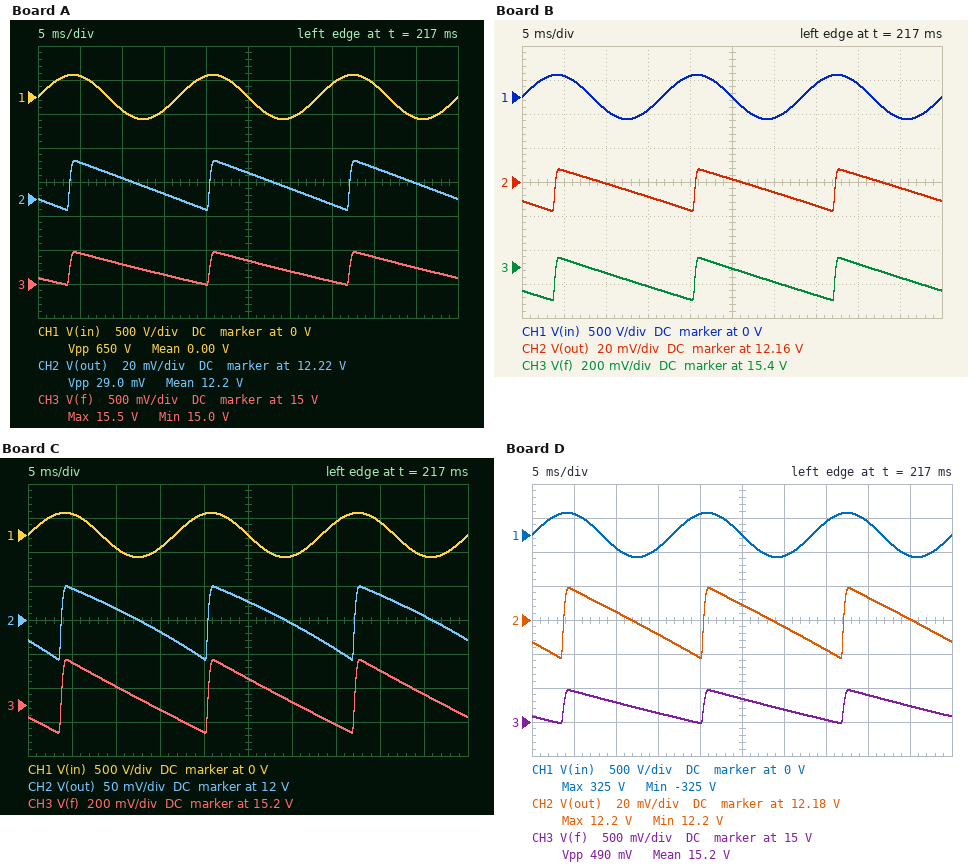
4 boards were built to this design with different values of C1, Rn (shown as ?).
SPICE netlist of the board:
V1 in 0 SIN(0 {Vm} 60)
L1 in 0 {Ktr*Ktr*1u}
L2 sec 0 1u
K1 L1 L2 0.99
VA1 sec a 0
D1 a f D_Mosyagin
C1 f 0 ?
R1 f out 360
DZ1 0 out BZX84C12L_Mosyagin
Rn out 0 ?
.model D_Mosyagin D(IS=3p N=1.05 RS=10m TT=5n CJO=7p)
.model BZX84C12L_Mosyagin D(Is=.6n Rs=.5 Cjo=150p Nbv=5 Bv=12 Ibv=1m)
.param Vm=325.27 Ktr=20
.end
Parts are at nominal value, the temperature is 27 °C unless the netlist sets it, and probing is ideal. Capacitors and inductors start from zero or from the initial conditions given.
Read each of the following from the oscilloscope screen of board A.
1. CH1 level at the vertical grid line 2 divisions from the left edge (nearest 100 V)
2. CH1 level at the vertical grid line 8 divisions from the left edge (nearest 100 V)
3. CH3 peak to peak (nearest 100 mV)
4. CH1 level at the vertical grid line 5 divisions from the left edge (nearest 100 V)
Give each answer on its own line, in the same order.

-200 V
200 V
500 mV
0 V
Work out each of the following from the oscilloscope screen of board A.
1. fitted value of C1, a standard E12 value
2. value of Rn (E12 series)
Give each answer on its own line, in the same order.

270 µF
4.7 kΩ
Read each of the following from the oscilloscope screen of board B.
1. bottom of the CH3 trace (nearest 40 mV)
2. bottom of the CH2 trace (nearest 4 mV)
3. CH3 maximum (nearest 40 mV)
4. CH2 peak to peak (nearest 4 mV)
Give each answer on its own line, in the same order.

15.20 V
12.144 V
15.44 V
24 mV
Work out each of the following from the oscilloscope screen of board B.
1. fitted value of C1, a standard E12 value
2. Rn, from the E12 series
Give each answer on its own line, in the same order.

560 µF
2.2 kΩ
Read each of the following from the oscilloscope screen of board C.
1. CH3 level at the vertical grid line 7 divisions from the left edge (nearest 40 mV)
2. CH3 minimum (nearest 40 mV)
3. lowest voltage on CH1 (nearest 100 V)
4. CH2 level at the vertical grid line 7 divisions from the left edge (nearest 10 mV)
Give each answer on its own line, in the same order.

15.08 V
15.04 V
-300 V
11.96 V
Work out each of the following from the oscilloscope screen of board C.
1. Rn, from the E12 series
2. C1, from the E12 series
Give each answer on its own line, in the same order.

1.5 kΩ
330 µF
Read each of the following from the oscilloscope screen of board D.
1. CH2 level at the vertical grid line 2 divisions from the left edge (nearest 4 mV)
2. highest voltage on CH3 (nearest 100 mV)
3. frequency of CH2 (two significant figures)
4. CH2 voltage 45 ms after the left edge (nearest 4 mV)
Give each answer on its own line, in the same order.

12.184 V
15.5 V
60 Hz
12.180 V
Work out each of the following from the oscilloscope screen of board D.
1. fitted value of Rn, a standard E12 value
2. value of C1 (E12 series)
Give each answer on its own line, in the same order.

2.7 kΩ
270 µF
